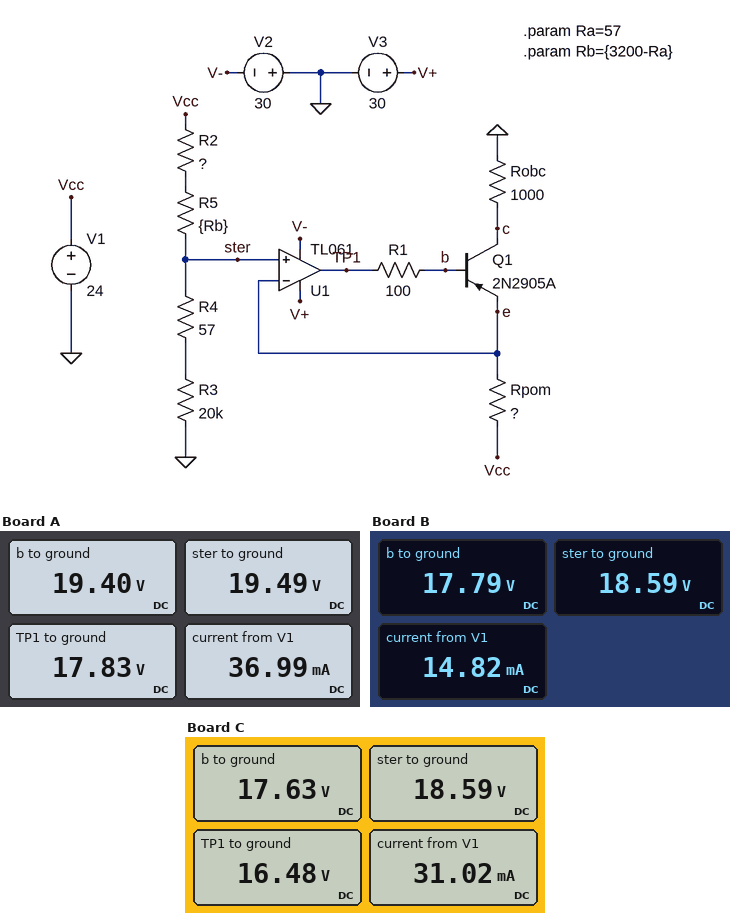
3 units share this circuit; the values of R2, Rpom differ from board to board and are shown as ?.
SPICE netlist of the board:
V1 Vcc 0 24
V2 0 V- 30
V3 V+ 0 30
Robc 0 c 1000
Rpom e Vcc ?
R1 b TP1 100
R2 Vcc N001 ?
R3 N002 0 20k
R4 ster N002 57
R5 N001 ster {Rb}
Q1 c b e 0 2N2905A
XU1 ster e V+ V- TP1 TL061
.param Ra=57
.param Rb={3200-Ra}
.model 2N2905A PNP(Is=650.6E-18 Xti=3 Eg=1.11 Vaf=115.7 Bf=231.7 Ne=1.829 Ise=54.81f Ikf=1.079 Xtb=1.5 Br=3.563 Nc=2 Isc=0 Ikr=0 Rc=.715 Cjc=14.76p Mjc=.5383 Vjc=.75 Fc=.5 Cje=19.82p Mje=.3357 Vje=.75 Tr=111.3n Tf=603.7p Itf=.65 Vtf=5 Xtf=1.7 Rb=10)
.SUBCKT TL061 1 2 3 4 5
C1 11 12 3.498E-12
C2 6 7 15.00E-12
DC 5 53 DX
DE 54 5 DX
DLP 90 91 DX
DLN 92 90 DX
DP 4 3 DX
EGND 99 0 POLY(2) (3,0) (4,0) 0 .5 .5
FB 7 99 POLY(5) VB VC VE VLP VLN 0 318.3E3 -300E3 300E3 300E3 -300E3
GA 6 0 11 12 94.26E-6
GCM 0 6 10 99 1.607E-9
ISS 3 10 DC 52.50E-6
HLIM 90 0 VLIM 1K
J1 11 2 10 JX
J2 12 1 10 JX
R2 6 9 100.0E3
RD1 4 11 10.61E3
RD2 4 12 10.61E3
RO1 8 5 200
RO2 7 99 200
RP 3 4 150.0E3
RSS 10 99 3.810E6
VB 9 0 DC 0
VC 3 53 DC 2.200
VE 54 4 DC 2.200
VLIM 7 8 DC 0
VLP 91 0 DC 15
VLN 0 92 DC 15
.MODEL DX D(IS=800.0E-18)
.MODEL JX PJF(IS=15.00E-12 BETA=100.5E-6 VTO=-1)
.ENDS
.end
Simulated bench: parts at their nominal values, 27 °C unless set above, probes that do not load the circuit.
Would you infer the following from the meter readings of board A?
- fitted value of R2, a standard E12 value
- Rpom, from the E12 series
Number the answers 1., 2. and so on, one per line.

1. 1.5 kΩ
2. 100 Ω
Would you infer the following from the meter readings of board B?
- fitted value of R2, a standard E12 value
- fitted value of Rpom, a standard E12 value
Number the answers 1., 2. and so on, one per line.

1. 2.7 kΩ
2. 390 Ω
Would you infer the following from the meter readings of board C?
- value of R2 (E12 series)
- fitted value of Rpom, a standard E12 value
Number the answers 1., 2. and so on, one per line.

1. 2.7 kΩ
2. 180 Ω
